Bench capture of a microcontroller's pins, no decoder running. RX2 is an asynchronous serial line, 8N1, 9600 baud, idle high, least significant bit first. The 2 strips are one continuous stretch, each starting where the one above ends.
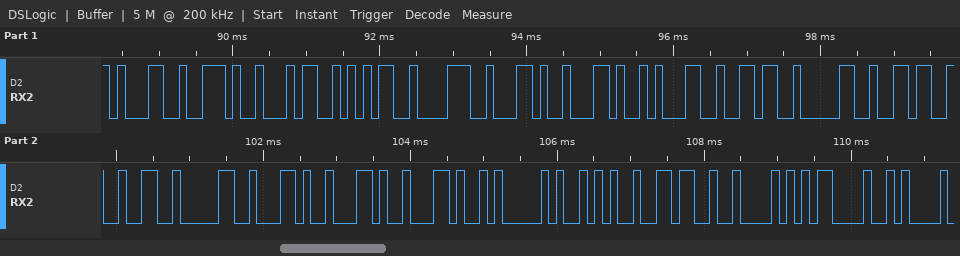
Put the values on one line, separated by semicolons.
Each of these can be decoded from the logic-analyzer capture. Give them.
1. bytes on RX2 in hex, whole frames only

0x31 0x2E 0x34 0x35 0x38 0x2C 0x2C 0x31 0x36 0x30 0x36 0x32 0x30 0x2C 0x2C 0x2C 0x41 0x2A 0x36 0x42 0x0D 0x0A
